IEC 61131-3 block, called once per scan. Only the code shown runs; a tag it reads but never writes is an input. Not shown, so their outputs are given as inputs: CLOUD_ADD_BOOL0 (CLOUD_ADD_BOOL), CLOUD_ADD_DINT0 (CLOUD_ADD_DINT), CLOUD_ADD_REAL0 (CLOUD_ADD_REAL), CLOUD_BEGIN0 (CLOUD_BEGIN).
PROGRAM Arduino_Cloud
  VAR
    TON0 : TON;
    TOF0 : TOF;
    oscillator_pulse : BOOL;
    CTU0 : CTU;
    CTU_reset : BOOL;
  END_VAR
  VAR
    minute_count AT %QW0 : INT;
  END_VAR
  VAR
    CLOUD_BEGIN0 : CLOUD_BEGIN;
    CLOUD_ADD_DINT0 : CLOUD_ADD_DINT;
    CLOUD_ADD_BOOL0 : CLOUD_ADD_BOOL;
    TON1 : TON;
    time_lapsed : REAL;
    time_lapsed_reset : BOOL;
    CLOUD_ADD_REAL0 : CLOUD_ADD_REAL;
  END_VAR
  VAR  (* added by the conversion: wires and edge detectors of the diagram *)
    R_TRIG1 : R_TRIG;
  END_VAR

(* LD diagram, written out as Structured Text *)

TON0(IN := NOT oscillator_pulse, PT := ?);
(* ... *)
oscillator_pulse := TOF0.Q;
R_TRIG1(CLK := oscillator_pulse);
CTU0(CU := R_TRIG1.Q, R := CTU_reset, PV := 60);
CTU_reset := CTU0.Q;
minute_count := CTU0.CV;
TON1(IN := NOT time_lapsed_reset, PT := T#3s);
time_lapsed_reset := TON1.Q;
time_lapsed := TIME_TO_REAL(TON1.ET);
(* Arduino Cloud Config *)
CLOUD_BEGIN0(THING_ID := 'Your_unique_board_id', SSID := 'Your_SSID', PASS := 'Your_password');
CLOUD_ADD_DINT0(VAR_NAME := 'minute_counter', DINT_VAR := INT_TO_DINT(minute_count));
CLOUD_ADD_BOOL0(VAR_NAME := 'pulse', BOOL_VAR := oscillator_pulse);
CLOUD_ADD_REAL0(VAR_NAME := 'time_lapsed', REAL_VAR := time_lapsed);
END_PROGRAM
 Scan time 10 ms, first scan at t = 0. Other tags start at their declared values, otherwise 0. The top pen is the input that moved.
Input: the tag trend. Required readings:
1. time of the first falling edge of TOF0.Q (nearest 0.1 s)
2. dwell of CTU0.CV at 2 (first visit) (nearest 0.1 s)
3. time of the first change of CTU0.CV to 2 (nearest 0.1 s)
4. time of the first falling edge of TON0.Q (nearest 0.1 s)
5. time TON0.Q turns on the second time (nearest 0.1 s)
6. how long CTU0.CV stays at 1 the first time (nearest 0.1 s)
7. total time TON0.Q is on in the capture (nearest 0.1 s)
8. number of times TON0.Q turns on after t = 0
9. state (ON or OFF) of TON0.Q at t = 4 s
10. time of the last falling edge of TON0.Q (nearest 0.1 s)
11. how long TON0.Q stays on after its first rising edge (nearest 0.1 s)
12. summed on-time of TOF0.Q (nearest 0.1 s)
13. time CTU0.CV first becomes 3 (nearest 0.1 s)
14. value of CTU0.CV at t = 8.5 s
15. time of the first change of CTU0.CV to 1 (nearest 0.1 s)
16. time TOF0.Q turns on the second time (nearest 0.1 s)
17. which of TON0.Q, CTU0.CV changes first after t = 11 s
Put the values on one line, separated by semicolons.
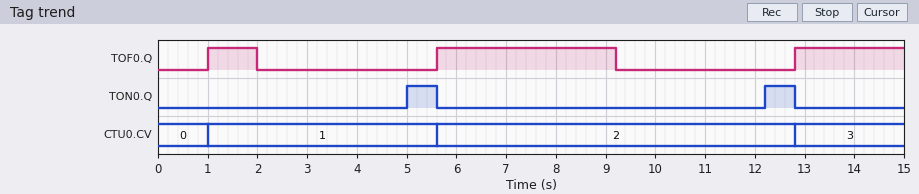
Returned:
2.0 s; 7.2 s; 5.6 s; 5.6 s; 12.2 s; 4.6 s; 1.2 s; 2; OFF; 12.8 s; 0.6 s; 6.8 s; 12.8 s; 2; 1.0 s; 5.6 s; TON0.Q
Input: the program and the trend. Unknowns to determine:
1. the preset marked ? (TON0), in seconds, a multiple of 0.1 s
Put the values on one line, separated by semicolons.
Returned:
3.0 s
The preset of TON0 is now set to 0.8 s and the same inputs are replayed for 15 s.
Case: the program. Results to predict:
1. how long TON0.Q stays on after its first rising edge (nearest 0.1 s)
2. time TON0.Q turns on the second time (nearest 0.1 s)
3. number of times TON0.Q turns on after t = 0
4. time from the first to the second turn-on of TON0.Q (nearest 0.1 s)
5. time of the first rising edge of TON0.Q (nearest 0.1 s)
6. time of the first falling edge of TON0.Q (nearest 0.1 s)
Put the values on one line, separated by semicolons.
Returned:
0.2 s; 2.8 s; 3; 2.0 s; 0.8 s; 1.0 s
